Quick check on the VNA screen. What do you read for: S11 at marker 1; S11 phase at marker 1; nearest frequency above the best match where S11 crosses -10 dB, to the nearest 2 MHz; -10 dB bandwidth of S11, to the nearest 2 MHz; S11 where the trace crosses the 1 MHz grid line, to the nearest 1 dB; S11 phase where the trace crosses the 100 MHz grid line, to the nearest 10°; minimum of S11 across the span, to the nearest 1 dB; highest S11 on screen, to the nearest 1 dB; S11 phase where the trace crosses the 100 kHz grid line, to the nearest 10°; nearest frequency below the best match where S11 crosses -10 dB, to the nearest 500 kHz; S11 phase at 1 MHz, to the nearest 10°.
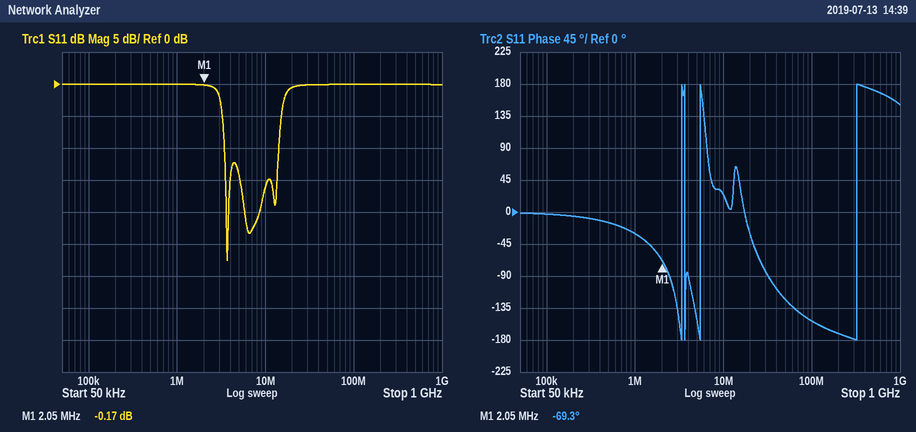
-0.17 dB
-69.3°
14 MHz
10 MHz
0 dB
-150°
-28 dB
0 dB
0°
3.5 MHz
-30°
